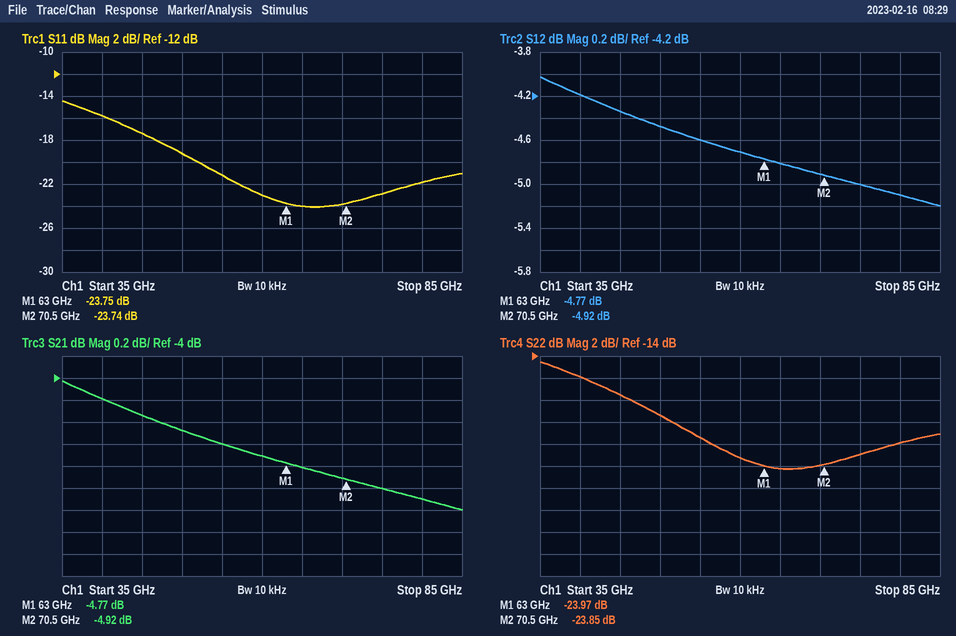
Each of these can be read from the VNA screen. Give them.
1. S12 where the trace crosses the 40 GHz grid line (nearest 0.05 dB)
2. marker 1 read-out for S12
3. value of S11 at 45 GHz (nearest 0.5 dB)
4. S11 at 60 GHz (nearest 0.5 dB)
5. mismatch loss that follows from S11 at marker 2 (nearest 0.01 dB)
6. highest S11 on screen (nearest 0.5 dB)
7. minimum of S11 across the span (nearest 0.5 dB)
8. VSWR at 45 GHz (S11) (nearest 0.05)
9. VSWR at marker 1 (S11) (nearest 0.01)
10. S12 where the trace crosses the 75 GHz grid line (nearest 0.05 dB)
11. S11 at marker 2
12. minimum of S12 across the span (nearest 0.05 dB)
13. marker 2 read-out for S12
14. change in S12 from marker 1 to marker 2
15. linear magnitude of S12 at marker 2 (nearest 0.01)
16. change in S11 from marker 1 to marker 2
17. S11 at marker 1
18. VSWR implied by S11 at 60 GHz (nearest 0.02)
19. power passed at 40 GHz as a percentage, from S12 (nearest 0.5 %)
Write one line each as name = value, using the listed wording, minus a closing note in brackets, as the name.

S12 where the trace crosses the 40 GHz grid line = -4.20 dB
marker 1 read-out for S12 = -4.77 dB
value of S11 at 45 GHz = -17.5 dB
S11 at 60 GHz = -23.0 dB
mismatch loss that follows from S11 at marker 2 = 0.02 dB
highest S11 on screen = -14.5 dB
minimum of S11 across the span = -24.0 dB
VSWR at 45 GHz (S11) = 1.30
VSWR at marker 1 (S11) = 1.14
S12 where the trace crosses the 75 GHz grid line = -5.00 dB
S11 at marker 2 = -23.74 dB
minimum of S12 across the span = -5.20 dB
marker 2 read-out for S12 = -4.92 dB
change in S12 from marker 1 to marker 2 = -0.15 dB
linear magnitude of S12 at marker 2 = 0.57
change in S11 from marker 1 to marker 2 = 0.01 dB
S11 at marker 1 = -23.75 dB
VSWR implied by S11 at 60 GHz = 1.16
power passed at 40 GHz as a percentage, from S12 = 38.0 %
